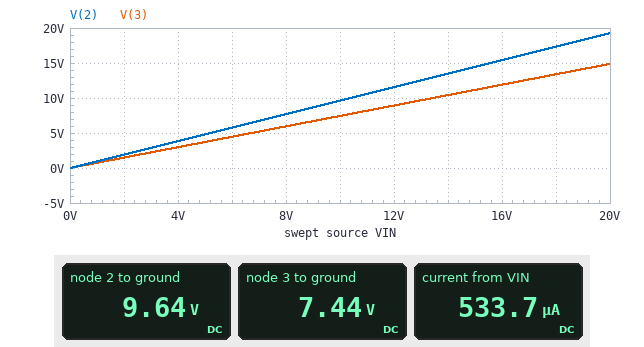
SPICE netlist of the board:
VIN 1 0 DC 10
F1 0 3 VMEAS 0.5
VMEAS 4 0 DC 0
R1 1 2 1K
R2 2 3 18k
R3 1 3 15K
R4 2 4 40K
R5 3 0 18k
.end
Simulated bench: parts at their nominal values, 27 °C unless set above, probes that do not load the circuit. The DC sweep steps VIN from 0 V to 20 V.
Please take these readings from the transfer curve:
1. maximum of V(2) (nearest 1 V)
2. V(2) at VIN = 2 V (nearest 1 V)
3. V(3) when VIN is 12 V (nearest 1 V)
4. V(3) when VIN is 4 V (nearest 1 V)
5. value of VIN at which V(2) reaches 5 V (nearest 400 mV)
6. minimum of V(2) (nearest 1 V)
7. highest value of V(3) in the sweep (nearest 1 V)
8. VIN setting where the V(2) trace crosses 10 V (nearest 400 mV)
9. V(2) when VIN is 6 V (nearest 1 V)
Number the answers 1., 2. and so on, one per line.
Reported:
1. 19 V
2. 2 V
3. 9 V
4. 3 V
5. 5.2 V
6. 0 V
7. 15 V
8. 10.4 V
9. 6 V
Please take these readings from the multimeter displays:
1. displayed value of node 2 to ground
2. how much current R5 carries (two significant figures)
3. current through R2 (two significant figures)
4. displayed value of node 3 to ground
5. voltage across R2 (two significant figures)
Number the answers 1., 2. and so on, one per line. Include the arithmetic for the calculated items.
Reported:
1. 9.64 V
2. (7.44 V) / 18 kΩ = 410 µA
3. (9.64 V - 7.44 V) / 18 kΩ = 120 µA
4. 7.44 V
5. 9.64 V - 7.44 V = 2.2 V
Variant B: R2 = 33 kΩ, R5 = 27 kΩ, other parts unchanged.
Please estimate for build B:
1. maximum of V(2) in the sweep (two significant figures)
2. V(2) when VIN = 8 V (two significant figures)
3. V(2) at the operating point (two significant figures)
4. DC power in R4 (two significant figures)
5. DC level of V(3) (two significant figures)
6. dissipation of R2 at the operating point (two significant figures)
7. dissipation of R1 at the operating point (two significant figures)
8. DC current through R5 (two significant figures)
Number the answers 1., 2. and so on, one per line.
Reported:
1. 19 V
2. 7.8 V
3. 9.7 V
4. 2.4 mW
5. 8.1 V
6. 81 µW
7. 85 µW
8. 300 µA
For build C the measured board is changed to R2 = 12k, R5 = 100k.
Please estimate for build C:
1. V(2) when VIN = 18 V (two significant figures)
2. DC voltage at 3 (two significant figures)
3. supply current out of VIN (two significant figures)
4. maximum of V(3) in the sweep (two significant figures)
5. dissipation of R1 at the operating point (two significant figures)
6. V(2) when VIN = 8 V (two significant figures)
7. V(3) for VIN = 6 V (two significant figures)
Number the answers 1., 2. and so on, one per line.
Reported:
1. 18 V
2. 10 V
3. 220 µA
4. 20 V
5. 50 µW
6. 7.8 V
7. 6.0 V
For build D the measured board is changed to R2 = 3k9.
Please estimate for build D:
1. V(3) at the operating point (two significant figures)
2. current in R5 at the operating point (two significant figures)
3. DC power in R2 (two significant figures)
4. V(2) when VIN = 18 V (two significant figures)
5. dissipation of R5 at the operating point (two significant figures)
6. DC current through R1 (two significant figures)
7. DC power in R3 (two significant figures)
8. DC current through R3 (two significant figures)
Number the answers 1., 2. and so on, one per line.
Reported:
1. 8.5 V
2. 470 µA
3. 250 µW
4. 17 V
5. 4.0 mW
6. 490 µA
7. 150 µW
8. 99 µA
